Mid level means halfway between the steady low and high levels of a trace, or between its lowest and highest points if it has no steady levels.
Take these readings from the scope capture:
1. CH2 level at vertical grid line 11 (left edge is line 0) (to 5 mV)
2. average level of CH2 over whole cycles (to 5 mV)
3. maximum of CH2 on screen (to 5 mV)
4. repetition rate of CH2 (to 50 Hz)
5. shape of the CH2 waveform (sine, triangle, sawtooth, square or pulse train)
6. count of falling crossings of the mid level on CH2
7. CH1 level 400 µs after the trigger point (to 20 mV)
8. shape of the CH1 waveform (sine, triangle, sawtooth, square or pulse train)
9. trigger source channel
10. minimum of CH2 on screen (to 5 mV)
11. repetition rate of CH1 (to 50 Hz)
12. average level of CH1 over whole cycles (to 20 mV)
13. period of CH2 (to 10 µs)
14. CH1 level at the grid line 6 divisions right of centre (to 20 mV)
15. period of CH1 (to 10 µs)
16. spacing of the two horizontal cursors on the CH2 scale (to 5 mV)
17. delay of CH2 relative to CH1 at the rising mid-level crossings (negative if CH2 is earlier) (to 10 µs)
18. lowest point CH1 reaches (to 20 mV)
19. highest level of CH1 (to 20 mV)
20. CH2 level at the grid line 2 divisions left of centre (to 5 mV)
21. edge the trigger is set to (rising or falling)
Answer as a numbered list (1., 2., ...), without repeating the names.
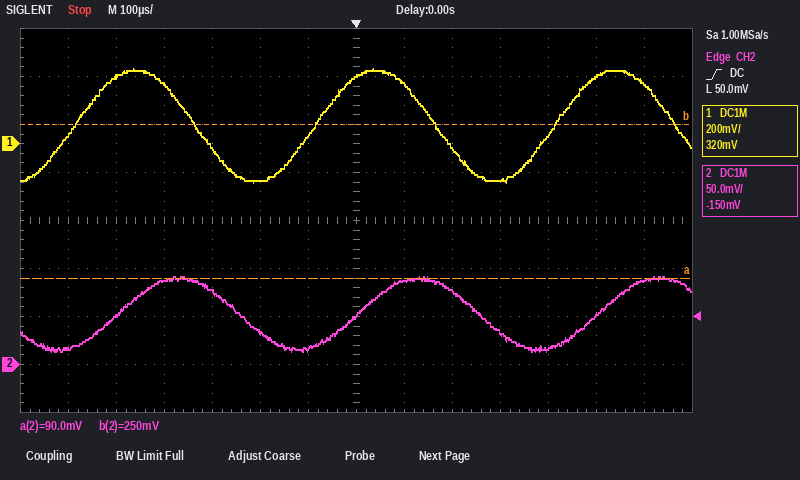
1. 15 mV
2. 55 mV
3. 90 mV
4. 2.00 kHz
5. sine
6. 2
7. 40 mV
8. sine
9. CH2
10. 15 mV
11. 2.00 kHz
12. 80 mV
13. 500 µs
14. 240 mV
15. 500 µs
16. 160 mV
17. +90 µs
18. -160 mV
19. 320 mV
20. 35 mV
21. rising
